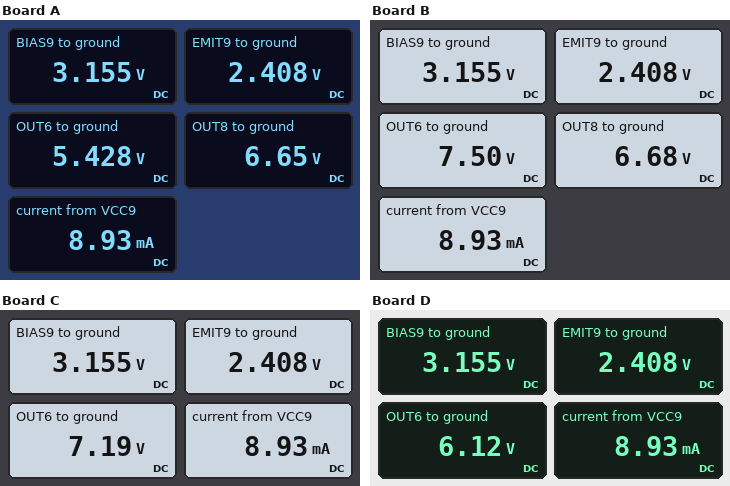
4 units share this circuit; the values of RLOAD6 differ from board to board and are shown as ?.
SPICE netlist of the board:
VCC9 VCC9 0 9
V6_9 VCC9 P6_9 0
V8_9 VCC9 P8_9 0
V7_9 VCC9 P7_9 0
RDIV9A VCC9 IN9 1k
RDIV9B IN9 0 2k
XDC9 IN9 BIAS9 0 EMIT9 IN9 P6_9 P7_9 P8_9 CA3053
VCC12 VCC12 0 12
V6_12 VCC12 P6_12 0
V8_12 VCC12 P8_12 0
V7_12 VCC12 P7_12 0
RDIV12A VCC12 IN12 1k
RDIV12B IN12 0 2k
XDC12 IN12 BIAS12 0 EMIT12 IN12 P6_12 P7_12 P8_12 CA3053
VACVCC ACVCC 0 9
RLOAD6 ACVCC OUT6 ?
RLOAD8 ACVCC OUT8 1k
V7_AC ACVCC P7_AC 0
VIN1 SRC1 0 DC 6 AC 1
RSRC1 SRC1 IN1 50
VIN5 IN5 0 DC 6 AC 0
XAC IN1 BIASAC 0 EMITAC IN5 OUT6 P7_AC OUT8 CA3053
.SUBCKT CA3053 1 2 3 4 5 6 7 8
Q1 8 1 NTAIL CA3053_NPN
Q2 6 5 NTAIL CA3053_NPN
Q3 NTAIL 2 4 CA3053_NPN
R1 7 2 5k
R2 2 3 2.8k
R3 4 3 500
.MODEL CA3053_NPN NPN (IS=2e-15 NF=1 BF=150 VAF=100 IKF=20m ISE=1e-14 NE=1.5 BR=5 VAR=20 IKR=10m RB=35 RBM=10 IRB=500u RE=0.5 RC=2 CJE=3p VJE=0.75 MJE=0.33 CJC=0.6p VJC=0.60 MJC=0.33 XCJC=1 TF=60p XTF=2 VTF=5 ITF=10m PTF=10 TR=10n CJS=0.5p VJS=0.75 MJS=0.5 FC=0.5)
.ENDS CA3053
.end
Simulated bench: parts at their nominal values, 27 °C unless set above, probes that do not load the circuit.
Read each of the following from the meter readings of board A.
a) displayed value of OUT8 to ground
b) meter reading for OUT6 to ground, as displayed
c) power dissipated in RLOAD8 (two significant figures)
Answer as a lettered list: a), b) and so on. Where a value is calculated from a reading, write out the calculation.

a) 6.65 V
b) 5.428 V
c) (9 V - 6.65 V)^2 / 1 kΩ = 5.5 mW
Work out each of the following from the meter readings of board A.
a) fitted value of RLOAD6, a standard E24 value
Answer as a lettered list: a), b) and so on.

a) 1.5 kΩ
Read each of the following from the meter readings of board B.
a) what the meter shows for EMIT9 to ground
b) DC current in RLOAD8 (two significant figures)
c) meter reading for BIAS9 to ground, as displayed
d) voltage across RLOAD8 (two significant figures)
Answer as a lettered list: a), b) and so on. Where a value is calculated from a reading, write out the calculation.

a) 2.408 V
b) (9 V - 6.68 V) / 1 kΩ = 2.3 mA
c) 3.155 V
d) 9 V - 6.68 V = 2.3 V
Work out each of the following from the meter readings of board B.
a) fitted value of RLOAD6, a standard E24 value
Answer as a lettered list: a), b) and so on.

a) 620 Ω
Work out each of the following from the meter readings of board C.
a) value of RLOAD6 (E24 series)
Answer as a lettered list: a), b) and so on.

a) 750 Ω
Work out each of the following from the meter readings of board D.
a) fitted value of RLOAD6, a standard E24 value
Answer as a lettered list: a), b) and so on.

a) 1.2 kΩ
